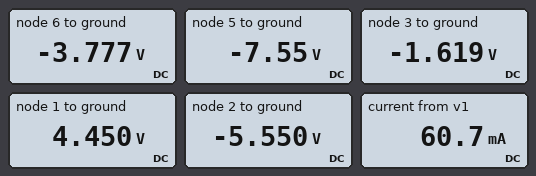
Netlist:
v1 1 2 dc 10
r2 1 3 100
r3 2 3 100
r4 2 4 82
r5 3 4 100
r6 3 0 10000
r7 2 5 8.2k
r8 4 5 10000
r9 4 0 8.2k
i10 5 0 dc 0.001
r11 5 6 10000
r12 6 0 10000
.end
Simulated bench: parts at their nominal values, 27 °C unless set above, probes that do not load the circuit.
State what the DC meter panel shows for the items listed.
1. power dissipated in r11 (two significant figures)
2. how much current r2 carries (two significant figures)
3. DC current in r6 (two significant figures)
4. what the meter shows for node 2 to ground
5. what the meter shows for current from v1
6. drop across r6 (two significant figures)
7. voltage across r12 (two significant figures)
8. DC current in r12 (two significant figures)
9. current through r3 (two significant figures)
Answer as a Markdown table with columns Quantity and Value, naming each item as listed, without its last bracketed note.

| Quantity | Value |
|---|---|
| power dissipated in r11 | 1.4 mW |
| how much current r2 carries | 61 mA |
| DC current in r6 | 160 µA |
| what the meter shows for node 2 to ground | -5.550 V |
| what the meter shows for current from v1 | 60.7 mA |
| drop across r6 | 1.6 V |
| voltage across r12 | 3.8 V |
| DC current in r12 | 380 µA |
| current through r3 | 39 mA |
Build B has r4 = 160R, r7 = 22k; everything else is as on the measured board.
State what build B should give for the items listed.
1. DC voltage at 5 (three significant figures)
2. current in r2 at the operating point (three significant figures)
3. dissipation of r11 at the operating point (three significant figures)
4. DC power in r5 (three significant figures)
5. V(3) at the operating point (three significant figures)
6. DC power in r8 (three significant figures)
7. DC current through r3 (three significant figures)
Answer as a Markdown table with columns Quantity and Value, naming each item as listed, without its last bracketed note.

| Quantity | Value |
|---|---|
| DC voltage at 5 | -8.23 V |
| current in r2 at the operating point | 58.0 mA |
| dissipation of r11 at the operating point | 1.69 mW |
| DC power in r5 | 26.2 mW |
| V(3) at the operating point | -1.76 V |
| DC power in r8 | 2.35 mW |
| DC current through r3 | 42.0 mA |
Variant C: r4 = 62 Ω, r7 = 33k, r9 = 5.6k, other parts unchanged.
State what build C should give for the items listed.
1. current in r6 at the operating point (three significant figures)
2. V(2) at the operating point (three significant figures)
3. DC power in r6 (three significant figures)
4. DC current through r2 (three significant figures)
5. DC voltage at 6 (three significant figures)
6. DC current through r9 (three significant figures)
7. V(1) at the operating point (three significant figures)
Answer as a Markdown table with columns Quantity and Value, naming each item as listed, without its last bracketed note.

| Quantity | Value |
|---|---|
| current in r6 at the operating point | 64.8 µA |
| V(2) at the operating point | -4.47 V |
| DC power in r6 | 42.0 µW |
| DC current through r2 | 61.8 mA |
| DC voltage at 6 | -3.98 V |
| DC current through r9 | 537 µA |
| V(1) at the operating point | 5.53 V |
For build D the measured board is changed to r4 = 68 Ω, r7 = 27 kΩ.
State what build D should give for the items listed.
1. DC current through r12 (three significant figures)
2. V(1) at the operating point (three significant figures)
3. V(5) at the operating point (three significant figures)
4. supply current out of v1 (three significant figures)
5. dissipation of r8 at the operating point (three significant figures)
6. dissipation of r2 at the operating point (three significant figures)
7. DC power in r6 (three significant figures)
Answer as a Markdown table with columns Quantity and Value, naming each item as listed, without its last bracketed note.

| Quantity | Value |
|---|---|
| DC current through r12 | 417 µA |
| V(1) at the operating point | 4.78 V |
| V(5) at the operating point | -8.34 V |
| supply current out of v1 | 61.4 mA |
| dissipation of r8 at the operating point | 2.19 mW |
| dissipation of r2 at the operating point | 377 mW |
| DC power in r6 | 186 µW |
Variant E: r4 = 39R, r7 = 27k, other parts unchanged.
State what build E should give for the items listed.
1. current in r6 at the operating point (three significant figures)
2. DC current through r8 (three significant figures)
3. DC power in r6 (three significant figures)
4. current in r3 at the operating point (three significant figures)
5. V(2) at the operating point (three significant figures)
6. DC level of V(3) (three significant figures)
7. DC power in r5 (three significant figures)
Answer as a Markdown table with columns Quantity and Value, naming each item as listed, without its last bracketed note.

| Quantity | Value |
|---|---|
| current in r6 at the operating point | 117 µA |
| DC current through r8 | 453 µA |
| DC power in r6 | 137 µW |
| current in r3 at the operating point | 36.8 mA |
| V(2) at the operating point | -4.85 V |
| DC level of V(3) | -1.17 V |
| DC power in r5 | 70.1 mW |
